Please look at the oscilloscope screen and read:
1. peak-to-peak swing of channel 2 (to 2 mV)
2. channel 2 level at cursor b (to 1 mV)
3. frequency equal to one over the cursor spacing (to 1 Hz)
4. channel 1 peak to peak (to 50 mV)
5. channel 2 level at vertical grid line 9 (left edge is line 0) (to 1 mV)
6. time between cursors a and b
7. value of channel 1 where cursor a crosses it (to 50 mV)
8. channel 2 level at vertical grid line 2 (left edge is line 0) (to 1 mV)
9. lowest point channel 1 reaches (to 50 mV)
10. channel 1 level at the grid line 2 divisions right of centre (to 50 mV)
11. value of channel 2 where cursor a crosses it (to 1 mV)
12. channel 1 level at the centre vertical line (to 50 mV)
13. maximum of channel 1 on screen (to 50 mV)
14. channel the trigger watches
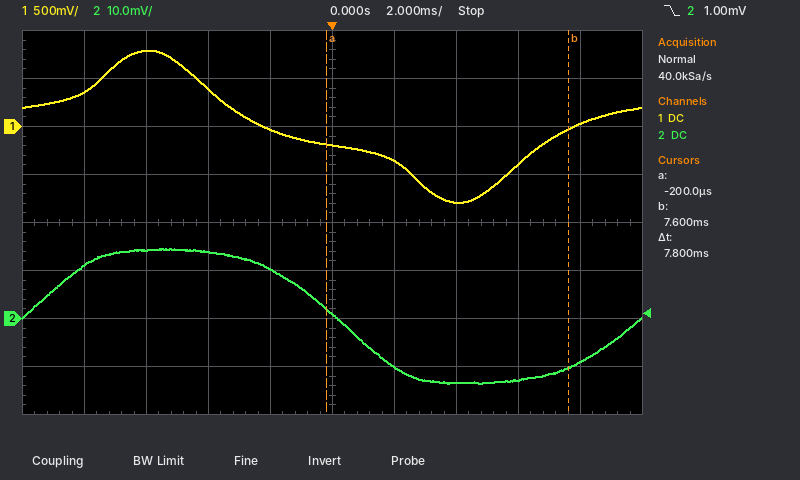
28 mV
-10 mV
128 Hz
1.60 V
-9 mV
7.8 ms
-200 mV
14 mV
-800 mV
-800 mV
2 mV
-200 mV
800 mV
channel 2
